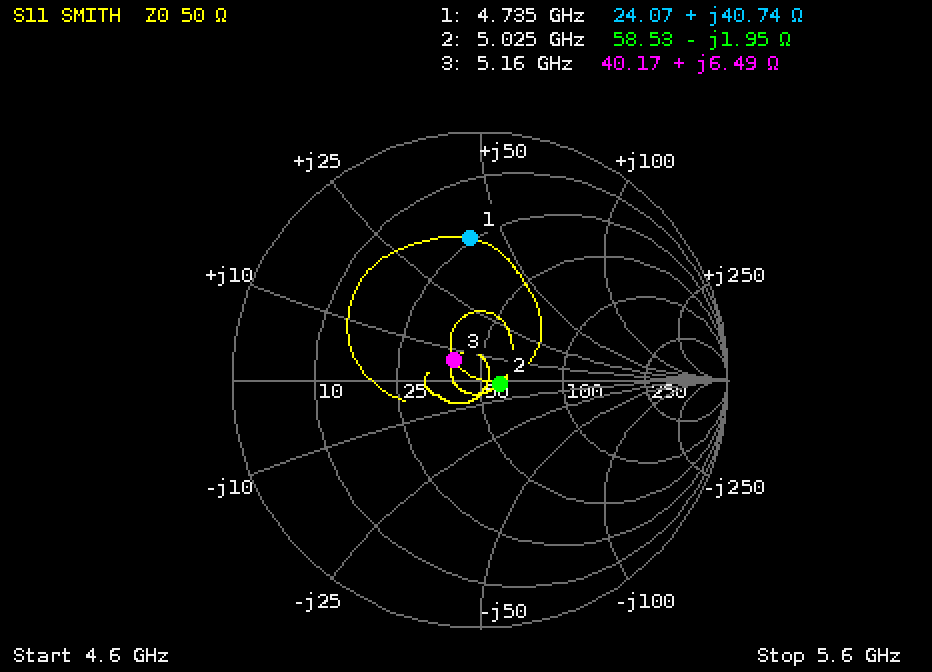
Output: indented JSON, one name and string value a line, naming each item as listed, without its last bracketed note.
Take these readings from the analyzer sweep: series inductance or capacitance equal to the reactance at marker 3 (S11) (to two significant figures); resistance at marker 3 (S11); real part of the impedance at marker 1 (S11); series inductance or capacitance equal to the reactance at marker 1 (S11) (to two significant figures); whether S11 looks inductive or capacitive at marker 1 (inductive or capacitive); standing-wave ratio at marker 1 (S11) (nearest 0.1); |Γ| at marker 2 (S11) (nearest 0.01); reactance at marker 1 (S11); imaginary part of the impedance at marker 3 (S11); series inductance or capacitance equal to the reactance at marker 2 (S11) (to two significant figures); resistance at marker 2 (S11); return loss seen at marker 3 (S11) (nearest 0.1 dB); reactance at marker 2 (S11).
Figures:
{
  "series inductance or capacitance equal to the reactance at marker 3 (S11)": "200 pH",
  "resistance at marker 3": "40.17 Ω",
  "real part of the impedance at marker 1": "24.07 Ω",
  "series inductance or capacitance equal to the reactance at marker 1 (S11)": "1.4 nH",
  "whether S11 looks inductive or capacitive at marker 1": "inductive",
  "standing-wave ratio at marker 1 (S11)": "3.7",
  "|Γ| at marker 2 (S11)": "0.08",
  "reactance at marker 1": "+40.74 Ω",
  "imaginary part of the impedance at marker 3": "+6.49 Ω",
  "series inductance or capacitance equal to the reactance at marker 2 (S11)": "16 pF",
  "resistance at marker 2": "58.53 Ω",
  "return loss seen at marker 3 (S11)": "17.7 dB",
  "reactance at marker 2": "-1.95 Ω"
}
